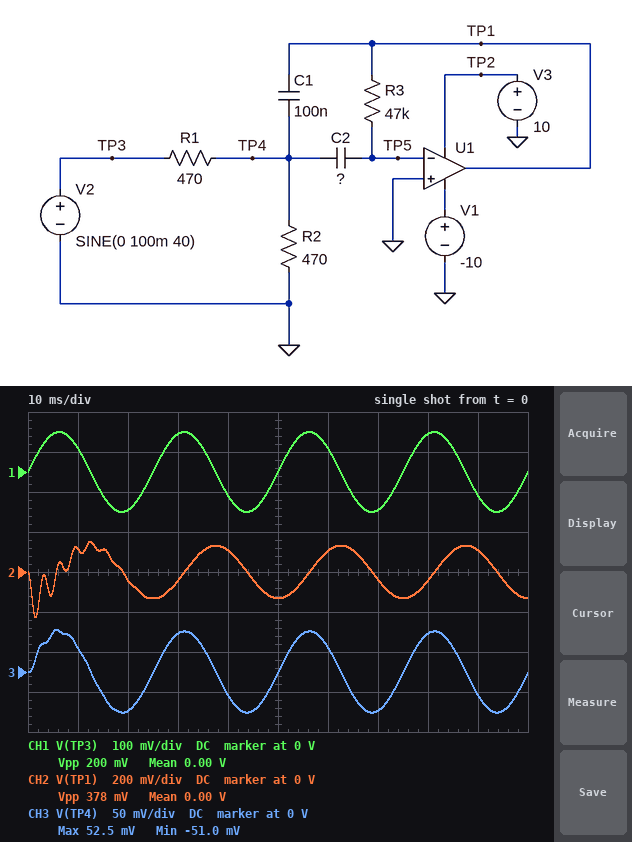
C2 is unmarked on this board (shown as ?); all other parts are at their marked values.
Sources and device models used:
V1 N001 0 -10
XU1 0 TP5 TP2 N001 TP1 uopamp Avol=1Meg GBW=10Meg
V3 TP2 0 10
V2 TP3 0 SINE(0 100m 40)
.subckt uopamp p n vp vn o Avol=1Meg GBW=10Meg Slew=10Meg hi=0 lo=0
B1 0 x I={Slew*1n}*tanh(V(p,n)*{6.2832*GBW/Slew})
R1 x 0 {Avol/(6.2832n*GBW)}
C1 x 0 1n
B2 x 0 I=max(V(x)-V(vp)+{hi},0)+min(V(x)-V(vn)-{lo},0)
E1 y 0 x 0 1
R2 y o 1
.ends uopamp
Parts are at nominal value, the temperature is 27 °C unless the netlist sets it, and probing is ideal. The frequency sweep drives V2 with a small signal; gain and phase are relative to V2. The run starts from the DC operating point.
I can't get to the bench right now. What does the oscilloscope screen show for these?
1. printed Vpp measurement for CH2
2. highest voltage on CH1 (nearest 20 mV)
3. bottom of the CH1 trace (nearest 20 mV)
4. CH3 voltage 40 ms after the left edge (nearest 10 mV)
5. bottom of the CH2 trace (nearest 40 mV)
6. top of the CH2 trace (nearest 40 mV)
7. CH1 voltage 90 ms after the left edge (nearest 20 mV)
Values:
378 mV
100 mV
-100 mV
-30 mV
-240 mV
160 mV
-60 mV
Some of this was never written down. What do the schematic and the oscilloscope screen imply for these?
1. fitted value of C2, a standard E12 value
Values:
220 nF
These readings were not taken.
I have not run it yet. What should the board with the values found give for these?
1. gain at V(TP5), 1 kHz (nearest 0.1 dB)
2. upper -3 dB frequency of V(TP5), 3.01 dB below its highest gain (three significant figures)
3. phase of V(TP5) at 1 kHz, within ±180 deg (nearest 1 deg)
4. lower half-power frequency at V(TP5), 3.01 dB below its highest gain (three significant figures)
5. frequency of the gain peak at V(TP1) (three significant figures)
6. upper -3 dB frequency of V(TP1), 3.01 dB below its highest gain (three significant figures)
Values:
-68.5 dB
353 Hz
3 deg
302 Hz
323 Hz
348 Hz
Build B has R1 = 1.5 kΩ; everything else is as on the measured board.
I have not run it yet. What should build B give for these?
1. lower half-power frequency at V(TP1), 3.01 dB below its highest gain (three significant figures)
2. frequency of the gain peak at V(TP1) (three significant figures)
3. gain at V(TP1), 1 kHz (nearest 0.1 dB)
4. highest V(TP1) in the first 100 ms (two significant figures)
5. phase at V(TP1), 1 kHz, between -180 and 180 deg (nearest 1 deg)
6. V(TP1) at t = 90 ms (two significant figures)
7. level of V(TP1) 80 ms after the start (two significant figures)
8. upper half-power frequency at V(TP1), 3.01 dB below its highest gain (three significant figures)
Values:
238 Hz
262 Hz
1.1 dB
72 mV
93 deg
52 mV
-21 mV
287 Hz
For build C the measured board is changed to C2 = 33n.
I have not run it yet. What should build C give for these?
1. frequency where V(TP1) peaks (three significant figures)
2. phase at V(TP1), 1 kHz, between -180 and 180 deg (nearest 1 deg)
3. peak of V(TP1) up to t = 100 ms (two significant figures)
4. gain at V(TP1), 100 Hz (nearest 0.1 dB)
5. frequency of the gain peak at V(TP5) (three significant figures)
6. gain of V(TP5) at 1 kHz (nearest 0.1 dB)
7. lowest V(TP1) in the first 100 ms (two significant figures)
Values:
833 Hz
114 deg
20 mV
-6.1 dB
839 Hz
-59.9 dB
-34 mV
